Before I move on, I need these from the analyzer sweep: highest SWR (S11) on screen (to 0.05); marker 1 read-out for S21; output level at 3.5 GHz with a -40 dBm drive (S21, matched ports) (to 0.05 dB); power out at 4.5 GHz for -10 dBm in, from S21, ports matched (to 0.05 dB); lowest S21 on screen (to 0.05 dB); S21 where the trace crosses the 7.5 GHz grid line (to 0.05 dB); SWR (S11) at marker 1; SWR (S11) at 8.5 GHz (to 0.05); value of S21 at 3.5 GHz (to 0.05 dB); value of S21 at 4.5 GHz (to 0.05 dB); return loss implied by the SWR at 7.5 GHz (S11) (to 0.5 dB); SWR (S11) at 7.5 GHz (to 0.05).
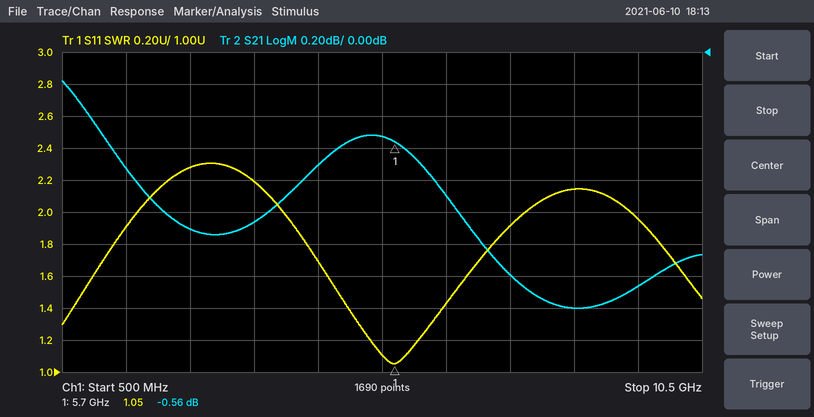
2.30
-0.56 dB
-41.05 dBm
-10.70 dBm
-1.60 dB
-1.40 dB
1.05
2.15
-1.05 dB
-0.70 dB
10.0 dB
1.90
